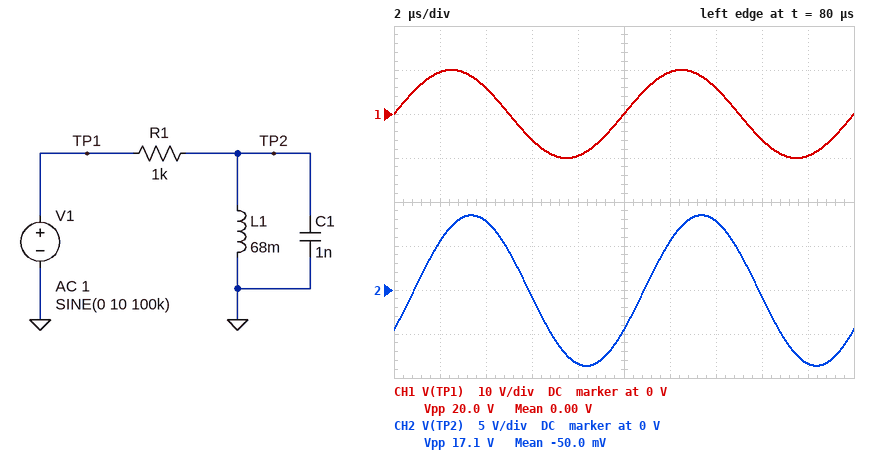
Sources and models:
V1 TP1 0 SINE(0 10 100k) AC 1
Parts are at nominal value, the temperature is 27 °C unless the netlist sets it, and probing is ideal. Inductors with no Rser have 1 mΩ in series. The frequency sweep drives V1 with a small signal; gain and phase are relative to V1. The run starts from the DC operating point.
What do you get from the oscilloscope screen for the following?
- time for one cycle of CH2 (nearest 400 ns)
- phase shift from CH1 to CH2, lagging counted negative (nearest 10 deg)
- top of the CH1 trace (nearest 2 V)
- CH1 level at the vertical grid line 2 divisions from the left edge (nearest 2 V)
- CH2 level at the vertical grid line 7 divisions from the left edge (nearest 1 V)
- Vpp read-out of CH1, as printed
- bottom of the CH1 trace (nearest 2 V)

10.0 µs
-30 deg
10 V
6 V
8 V
20.0 V
-10 V
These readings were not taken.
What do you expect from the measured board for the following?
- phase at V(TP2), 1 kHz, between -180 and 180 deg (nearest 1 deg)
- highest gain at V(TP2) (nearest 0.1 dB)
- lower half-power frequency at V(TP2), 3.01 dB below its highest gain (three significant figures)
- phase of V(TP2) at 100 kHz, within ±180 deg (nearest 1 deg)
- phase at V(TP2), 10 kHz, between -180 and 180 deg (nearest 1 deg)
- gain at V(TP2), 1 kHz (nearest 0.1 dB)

67 deg
0 dB
2.31 kHz
-31 deg
10 deg
-8.1 dB
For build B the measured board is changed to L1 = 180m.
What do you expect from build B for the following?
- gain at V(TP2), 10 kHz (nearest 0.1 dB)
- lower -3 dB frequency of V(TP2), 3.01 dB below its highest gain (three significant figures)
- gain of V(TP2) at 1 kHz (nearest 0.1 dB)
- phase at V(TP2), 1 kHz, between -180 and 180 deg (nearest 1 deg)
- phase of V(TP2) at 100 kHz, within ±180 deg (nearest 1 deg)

0 dB
879 Hz
-2.5 dB
41 deg
-32 deg
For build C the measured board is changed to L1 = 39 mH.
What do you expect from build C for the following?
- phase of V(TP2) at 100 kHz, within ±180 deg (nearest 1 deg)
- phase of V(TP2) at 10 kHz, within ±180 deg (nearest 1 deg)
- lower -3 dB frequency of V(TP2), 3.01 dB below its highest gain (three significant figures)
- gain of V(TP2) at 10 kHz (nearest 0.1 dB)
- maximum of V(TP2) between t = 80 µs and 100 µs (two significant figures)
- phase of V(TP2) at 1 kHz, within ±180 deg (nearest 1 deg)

-30 deg
19 deg
3.98 kHz
-0.5 dB
8.6 V
76 deg
